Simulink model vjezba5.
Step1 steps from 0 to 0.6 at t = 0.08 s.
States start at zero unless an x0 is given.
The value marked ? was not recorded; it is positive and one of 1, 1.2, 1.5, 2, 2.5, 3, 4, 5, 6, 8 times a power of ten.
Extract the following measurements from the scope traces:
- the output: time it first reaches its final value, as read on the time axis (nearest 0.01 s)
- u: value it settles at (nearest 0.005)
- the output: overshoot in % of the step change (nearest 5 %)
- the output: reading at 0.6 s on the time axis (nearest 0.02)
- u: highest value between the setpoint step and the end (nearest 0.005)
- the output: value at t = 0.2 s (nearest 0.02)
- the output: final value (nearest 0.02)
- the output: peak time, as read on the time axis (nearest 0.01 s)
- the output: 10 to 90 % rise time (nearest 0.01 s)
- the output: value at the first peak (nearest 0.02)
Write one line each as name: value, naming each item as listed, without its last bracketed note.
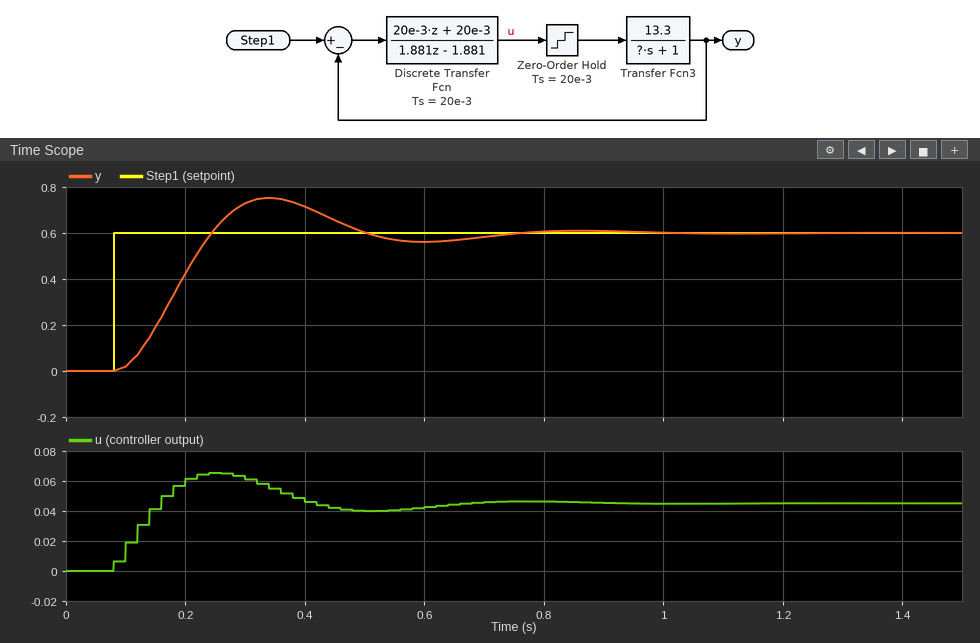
the output: time it first reaches its final value, as read on the time axis: 0.24 s
u: value it settles at: 0.045
the output: overshoot in % of the step change: 25 %
the output: reading at 0.6 s on the time axis: 0.56
u: highest value between the setpoint step and the end: 0.065
the output: value at t = 0.2 s: 0.42
the output: final value: 0.60
the output: peak time, as read on the time axis: 0.34 s
the output: 10 to 90 % rise time: 0.11 s
the output: value at the first peak: 0.76
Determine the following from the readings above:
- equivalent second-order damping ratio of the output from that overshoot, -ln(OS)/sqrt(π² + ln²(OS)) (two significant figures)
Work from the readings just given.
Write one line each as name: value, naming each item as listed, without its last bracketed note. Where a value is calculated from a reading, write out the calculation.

equivalent second-order damping ratio of the output from that overshoot, -ln(OS)/sqrt(π² + ln²(OS)): ln(0.25) = -1.386; 1.386 / sqrt(9.870 + 1.922) = 0.40
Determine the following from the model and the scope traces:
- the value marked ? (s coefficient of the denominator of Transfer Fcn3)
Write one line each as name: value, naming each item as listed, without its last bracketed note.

the value marked ?: 0.08
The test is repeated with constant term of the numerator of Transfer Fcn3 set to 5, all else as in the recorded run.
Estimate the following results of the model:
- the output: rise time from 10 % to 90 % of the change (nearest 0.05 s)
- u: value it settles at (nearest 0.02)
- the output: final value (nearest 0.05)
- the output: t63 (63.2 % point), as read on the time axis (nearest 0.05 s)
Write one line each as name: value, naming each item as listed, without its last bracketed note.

the output: rise time from 10 % to 90 % of the change: 0.25 s
u: value it settles at: 0.12
the output: final value: 0.60
the output: t63 (63.2 % point), as read on the time axis: 0.30 s
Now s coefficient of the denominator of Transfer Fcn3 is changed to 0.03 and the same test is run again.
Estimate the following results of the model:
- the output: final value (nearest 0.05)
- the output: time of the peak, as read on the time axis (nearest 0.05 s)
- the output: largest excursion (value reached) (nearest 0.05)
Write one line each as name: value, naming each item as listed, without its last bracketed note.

the output: final value: 0.60
the output: time of the peak, as read on the time axis: 0.30 s
the output: largest excursion (value reached): 0.65
